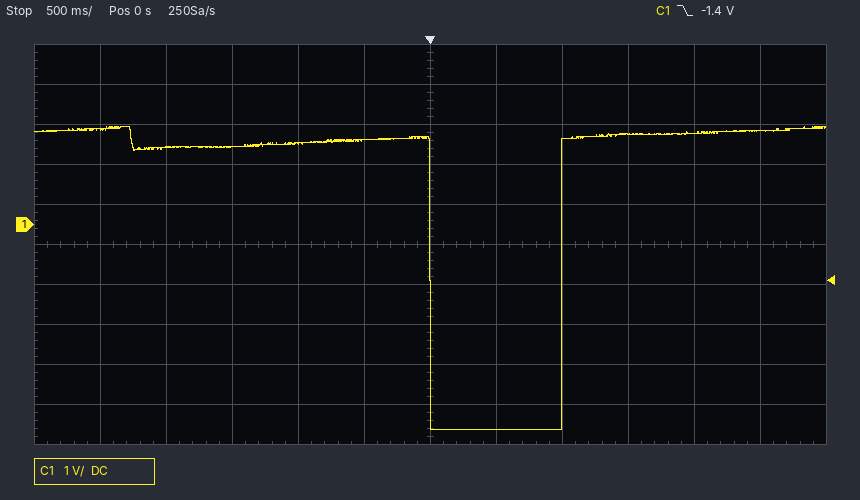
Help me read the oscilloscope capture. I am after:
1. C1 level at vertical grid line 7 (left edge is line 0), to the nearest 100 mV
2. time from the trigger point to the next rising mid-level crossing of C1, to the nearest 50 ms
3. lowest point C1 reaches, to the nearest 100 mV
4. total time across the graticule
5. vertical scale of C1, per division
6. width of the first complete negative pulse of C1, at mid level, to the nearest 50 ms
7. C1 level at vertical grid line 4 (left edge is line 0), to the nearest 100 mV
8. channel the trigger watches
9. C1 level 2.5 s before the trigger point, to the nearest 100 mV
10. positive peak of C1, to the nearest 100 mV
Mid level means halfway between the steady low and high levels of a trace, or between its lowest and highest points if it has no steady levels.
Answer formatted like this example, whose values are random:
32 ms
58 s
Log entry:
-5.1 V
1.00 s
-5.1 V
6 s
1 V
1.00 s
2.0 V
C1
2.4 V
2.4 V
